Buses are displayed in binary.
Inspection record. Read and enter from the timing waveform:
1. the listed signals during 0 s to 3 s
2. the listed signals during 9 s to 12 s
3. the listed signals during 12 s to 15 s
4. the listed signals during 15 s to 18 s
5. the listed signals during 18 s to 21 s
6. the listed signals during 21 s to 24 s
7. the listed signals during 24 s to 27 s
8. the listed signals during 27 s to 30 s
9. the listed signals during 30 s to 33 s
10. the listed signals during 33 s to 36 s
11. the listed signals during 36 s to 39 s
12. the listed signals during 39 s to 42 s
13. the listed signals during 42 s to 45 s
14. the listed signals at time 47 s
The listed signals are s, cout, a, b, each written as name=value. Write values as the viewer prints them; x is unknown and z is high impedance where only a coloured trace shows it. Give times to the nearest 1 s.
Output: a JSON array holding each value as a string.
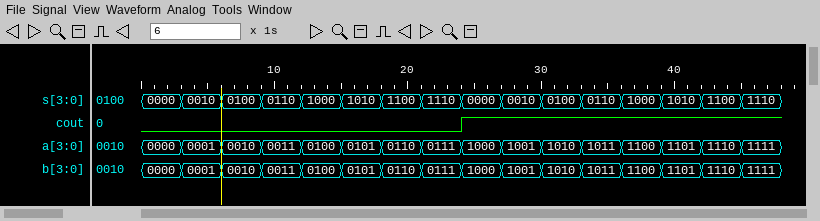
["s=0000, cout=0, a=0000, b=0000", "s=0110, cout=0, a=0011, b=0011", "s=1000, cout=0, a=0100, b=0100", "s=1010, cout=0, a=0101, b=0101", "s=1100, cout=0, a=0110, b=0110", "s=1110, cout=0, a=0111, b=0111", "s=0000, cout=1, a=1000, b=1000", "s=0010, cout=1, a=1001, b=1001", "s=0100, cout=1, a=1010, b=1010", "s=0110, cout=1, a=1011, b=1011", "s=1000, cout=1, a=1100, b=1100", "s=1010, cout=1, a=1101, b=1101", "s=1100, cout=1, a=1110, b=1110", "s=1110, cout=1, a=1111, b=1111"]
